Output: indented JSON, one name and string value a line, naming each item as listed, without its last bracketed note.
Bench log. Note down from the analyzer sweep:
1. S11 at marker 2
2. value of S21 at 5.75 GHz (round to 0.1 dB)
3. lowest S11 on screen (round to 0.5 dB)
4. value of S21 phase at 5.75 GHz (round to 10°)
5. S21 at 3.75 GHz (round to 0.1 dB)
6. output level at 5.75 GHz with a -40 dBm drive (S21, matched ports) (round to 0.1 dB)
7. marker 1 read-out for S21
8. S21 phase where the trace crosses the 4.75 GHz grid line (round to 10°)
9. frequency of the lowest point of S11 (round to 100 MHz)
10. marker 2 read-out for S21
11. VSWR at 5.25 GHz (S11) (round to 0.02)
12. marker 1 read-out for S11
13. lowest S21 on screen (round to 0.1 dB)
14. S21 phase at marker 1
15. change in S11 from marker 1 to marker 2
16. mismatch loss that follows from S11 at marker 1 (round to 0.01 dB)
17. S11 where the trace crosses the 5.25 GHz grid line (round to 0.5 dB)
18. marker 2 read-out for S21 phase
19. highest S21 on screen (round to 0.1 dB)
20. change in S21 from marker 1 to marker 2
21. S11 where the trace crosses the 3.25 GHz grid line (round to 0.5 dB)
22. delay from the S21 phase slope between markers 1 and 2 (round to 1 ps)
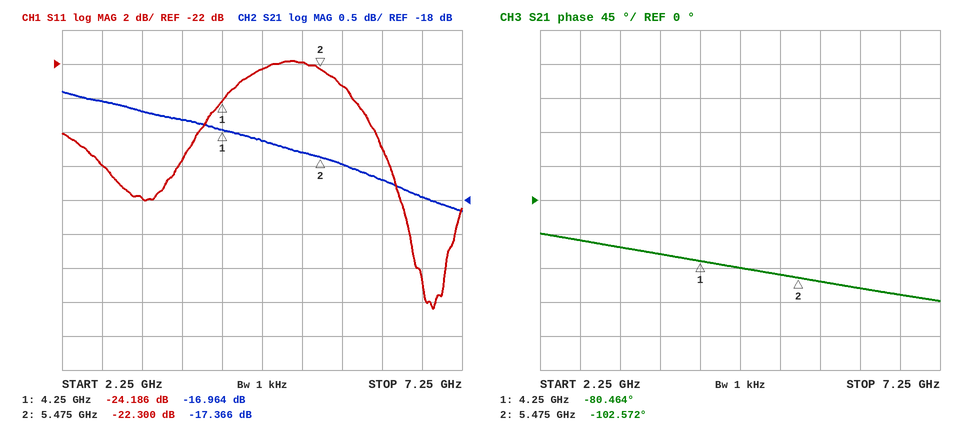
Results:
{
  "S11 at marker 2": "-22.300 dB",
  "value of S21 at 5.75 GHz": "-17.5 dB",
  "lowest S11 on screen": "-36.5 dB",
  "value of S21 phase at 5.75 GHz": "-110°",
  "S21 at 3.75 GHz": "-16.8 dB",
  "output level at 5.75 GHz with a -40 dBm drive (S21, matched ports)": "-57.5 dBm",
  "marker 1 read-out for S21": "-16.964 dB",
  "S21 phase where the trace crosses the 4.75 GHz grid line": "-90°",
  "frequency of the lowest point of S11": "6.9 GHz",
  "marker 2 read-out for S21": "-17.366 dB",
  "VSWR at 5.25 GHz (S11)": "1.18",
  "marker 1 read-out for S11": "-24.186 dB",
  "lowest S21 on screen": "-18.2 dB",
  "S21 phase at marker 1": "-80.464°",
  "change in S11 from marker 1 to marker 2": "1.886 dB",
  "mismatch loss that follows from S11 at marker 1": "0.02 dB",
  "S11 where the trace crosses the 5.25 GHz grid line": "-22.0 dB",
  "marker 2 read-out for S21 phase": "-102.572°",
  "highest S21 on screen": "-16.4 dB",
  "change in S21 from marker 1 to marker 2": "-0.402 dB",
  "S11 where the trace crosses the 3.25 GHz grid line": "-30.0 dB",
  "delay from the S21 phase slope between markers 1 and 2": "50 ps"
}
